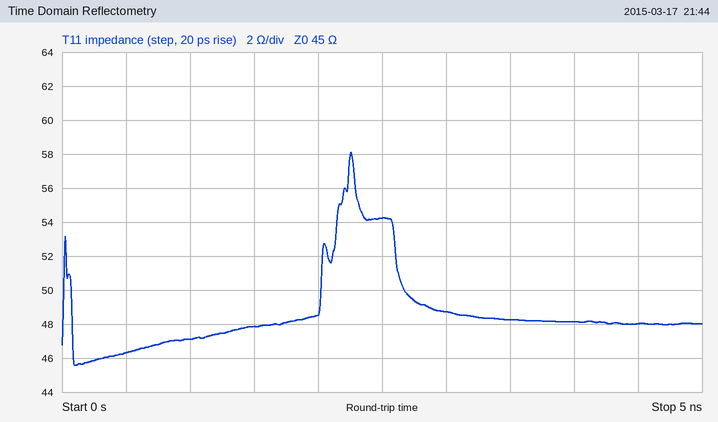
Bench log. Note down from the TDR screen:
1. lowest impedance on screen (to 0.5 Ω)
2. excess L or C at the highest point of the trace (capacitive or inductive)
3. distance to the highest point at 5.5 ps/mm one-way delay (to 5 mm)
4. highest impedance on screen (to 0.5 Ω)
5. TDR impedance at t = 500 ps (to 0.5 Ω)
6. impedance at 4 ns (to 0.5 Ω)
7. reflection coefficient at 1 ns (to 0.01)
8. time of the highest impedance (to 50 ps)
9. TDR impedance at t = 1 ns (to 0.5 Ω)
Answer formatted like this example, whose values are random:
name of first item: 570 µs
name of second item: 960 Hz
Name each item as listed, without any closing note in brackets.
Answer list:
lowest impedance on screen: 45.5 Ω
excess L or C at the highest point of the trace: inductive
distance to the highest point at 5.5 ps/mm one-way delay: 205 mm
highest impedance on screen: 58.0 Ω
TDR impedance at t = 500 ps: 46.5 Ω
impedance at 4 ns: 48.0 Ω
reflection coefficient at 1 ns: +0.02
time of the highest impedance: 2.25 ns
TDR impedance at t = 1 ns: 47.0 Ω
